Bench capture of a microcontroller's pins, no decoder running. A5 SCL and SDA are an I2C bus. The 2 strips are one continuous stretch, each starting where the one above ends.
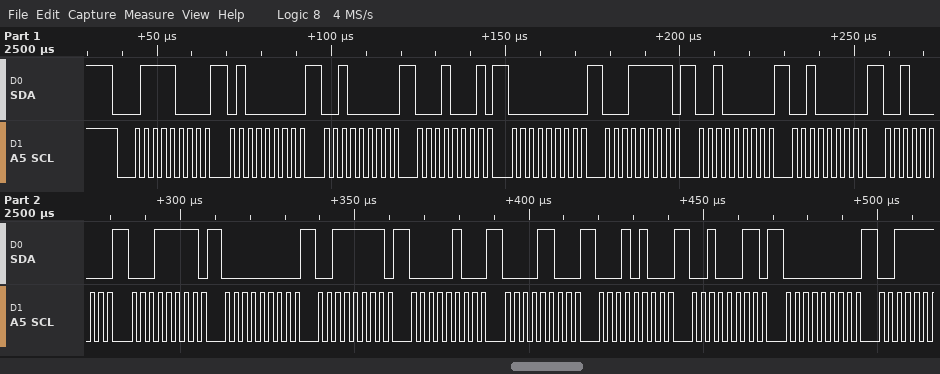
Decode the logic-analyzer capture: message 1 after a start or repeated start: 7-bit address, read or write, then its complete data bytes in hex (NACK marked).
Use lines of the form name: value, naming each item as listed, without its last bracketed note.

message 1 after a start or repeated start: 7-bit address, read or write, then its complete data bytes in hex: 0x3C write: 40 20 11 00 1F 20 20 20 1F 00 3F 04 0C 14 23 00
